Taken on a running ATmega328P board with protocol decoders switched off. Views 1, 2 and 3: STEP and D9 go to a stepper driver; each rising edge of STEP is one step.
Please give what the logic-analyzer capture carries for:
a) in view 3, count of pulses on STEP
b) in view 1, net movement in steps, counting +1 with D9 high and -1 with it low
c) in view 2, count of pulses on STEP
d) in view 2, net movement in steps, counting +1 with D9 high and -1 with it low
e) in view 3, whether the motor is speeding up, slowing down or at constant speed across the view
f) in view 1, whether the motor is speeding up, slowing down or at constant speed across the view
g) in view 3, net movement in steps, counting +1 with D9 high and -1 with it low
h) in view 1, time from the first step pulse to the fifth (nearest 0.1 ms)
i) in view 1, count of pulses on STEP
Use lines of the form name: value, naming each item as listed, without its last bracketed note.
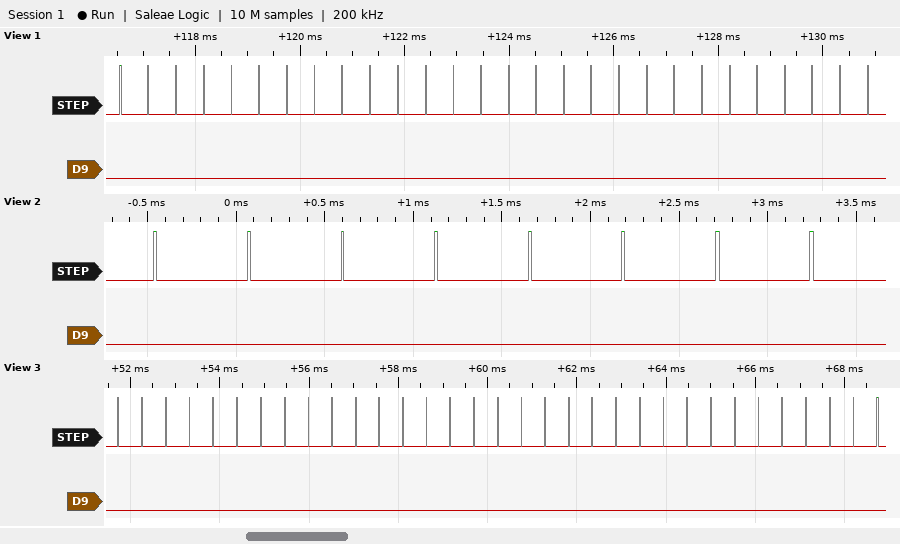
in view 3, count of pulses on STEP: 33
in view 1, net movement in steps, counting +1 with D9 high and -1 with it low: -28
in view 2, count of pulses on STEP: 8
in view 2, net movement in steps, counting +1 with D9 high and -1 with it low: -8
in view 3, whether the motor is speeding up, slowing down or at constant speed across the view: constant speed
in view 1, whether the motor is speeding up, slowing down or at constant speed across the view: constant speed
in view 3, net movement in steps, counting +1 with D9 high and -1 with it low: -33
in view 1, time from the first step pulse to the fifth: 2.1 ms
in view 1, count of pulses on STEP: 28
